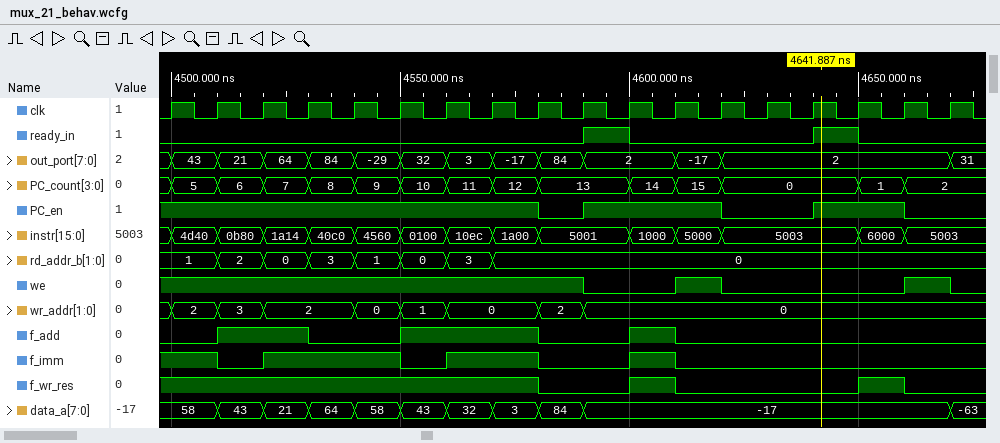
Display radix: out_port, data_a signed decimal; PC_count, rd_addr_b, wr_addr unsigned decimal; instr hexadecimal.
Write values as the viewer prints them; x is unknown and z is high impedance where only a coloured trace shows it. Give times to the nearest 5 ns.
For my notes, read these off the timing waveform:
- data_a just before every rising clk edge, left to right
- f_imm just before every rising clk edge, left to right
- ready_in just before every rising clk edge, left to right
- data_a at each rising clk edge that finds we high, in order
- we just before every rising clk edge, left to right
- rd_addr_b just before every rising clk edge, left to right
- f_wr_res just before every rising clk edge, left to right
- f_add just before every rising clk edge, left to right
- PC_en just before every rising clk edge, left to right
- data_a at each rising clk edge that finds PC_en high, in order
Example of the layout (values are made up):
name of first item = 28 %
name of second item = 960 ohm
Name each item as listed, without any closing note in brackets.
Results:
data_a just before every rising clk edge, left to right = 58, 58, 43, 21, 64, 58, 43, 32, 3, 84, -17, -17, -17, -17, -17, -17, -17, -17
f_imm just before every rising clk edge, left to right = 1 1 0 1 1 1 0 1 1 0 0 1 0 0 0 0 0 0
ready_in just before every rising clk edge, left to right = 0 0 0 0 0 0 0 0 0 0 1 0 0 0 0 1 0 0
data_a at each rising clk edge that finds we high, in order = 58, 58, 43, 21, 64, 58, 43, 32, 3, 84, -17, -17
we just before every rising clk edge, left to right = 1 1 1 1 1 1 1 1 1 1 0 0 1 0 0 0 0 1
rd_addr_b just before every rising clk edge, left to right = 1, 1, 2, 0, 3, 1, 0, 3, 0, 0, 0, 0, 0, 0, 0, 0, 0, 0
f_wr_res just before every rising clk edge, left to right = 1 1 1 1 1 1 1 1 1 0 0 1 0 0 0 0 1 0
f_add just before every rising clk edge, left to right = 0 0 1 1 0 0 1 1 1 0 0 1 0 0 0 0 0 0
PC_en just before every rising clk edge, left to right = 1 1 1 1 1 1 1 1 1 0 1 1 1 0 0 1 1 0
data_a at each rising clk edge that finds PC_en high, in order = 58, 58, 43, 21, 64, 58, 43, 32, 3, -17, -17, -17, -17, -17
